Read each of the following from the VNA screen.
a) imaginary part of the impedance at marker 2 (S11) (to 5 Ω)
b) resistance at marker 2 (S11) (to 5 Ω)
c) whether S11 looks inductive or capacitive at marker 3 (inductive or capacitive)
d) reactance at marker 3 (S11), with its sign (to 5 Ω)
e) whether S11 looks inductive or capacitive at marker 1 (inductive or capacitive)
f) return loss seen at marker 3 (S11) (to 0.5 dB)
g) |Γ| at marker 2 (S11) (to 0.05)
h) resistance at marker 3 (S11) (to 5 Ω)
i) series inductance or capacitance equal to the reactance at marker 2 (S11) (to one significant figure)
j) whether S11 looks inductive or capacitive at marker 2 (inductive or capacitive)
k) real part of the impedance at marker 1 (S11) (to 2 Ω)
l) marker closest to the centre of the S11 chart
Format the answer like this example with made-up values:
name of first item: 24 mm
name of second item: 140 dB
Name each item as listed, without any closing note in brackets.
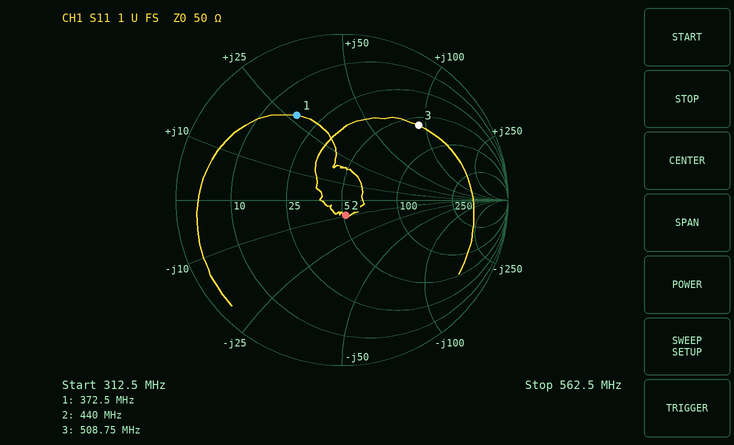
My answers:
imaginary part of the impedance at marker 2 (S11): -10 Ω
resistance at marker 2 (S11): 50 Ω
whether S11 looks inductive or capacitive at marker 3: inductive
reactance at marker 3 (S11), with its sign: +90 Ω
whether S11 looks inductive or capacitive at marker 1: inductive
return loss seen at marker 3 (S11): 4.0 dB
|Γ| at marker 2 (S11): 0.10
resistance at marker 3 (S11): 60 Ω
series inductance or capacitance equal to the reactance at marker 2 (S11): 40 pF
whether S11 looks inductive or capacitive at marker 2: capacitive
real part of the impedance at marker 1 (S11): 18 Ω
marker closest to the centre of the S11 chart: marker 2
